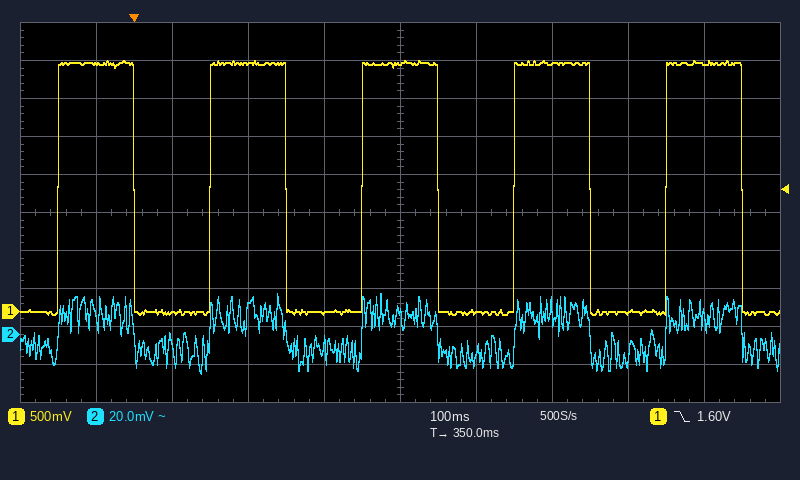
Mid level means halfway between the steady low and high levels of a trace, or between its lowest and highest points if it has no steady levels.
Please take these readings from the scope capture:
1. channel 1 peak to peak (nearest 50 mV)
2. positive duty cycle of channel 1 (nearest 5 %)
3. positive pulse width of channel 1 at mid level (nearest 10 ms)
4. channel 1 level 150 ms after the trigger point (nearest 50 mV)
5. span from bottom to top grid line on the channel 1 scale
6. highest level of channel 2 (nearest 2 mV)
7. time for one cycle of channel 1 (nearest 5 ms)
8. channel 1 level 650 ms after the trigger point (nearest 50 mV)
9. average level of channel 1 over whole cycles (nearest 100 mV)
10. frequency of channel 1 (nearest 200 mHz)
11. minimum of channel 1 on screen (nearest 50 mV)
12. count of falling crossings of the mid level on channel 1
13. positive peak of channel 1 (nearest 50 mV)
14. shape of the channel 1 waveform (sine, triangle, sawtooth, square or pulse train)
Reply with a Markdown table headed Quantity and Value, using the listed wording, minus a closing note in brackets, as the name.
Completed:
| Quantity | Value |
|---|---|
| channel 1 peak to peak | 3.35 V |
| positive duty cycle of channel 1 | 50 % |
| positive pulse width of channel 1 at mid level | 100 ms |
| channel 1 level 150 ms after the trigger point | 3.25 V |
| span from bottom to top grid line on the channel 1 scale | 5 V |
| highest level of channel 2 | 22 mV |
| time for one cycle of channel 1 | 200 ms |
| channel 1 level 650 ms after the trigger point | 0 mV |
| average level of channel 1 over whole cycles | 1.6 V |
| frequency of channel 1 | 5.0 Hz |
| minimum of channel 1 on screen | -50 mV |
| count of falling crossings of the mid level on channel 1 | 5 |
| positive peak of channel 1 | 3.30 V |
| shape of the channel 1 waveform | square |
